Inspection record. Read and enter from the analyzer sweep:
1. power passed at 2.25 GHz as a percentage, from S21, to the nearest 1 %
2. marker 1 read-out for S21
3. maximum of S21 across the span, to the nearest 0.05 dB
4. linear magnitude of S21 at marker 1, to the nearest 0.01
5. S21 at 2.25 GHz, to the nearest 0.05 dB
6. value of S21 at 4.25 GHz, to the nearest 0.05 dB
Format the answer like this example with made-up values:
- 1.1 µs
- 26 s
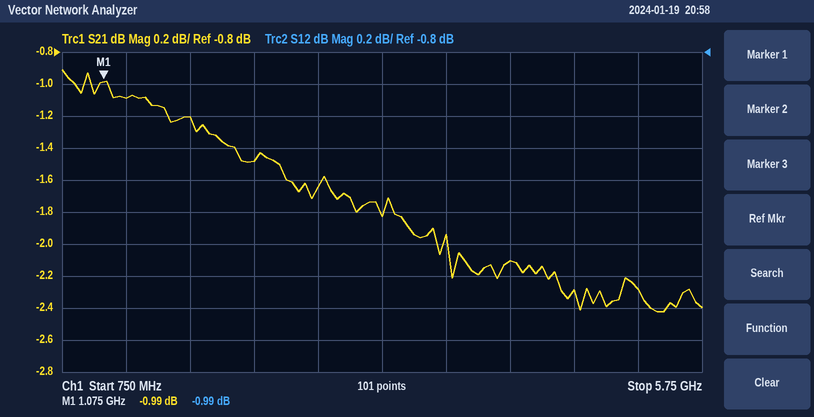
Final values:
- 71 %
- -0.99 dB
- -0.90 dB
- 0.89
- -1.50 dB
- -2.10 dB
